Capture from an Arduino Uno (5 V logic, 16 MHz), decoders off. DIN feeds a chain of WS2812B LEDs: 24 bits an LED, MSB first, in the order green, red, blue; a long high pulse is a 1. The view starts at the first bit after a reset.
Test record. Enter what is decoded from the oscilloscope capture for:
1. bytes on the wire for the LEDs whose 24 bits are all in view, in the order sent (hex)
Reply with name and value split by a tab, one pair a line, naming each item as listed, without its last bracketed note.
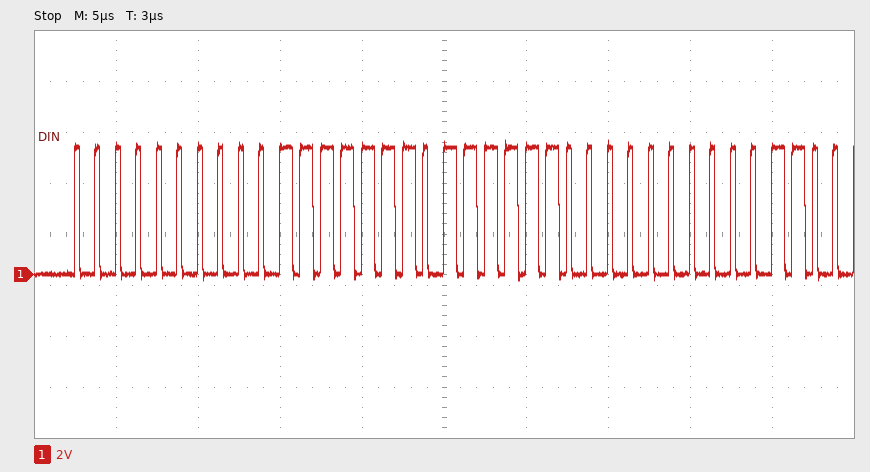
bytes on the wire for the LEDs whose 24 bits are all in view, in the order sent	00 3F BF
